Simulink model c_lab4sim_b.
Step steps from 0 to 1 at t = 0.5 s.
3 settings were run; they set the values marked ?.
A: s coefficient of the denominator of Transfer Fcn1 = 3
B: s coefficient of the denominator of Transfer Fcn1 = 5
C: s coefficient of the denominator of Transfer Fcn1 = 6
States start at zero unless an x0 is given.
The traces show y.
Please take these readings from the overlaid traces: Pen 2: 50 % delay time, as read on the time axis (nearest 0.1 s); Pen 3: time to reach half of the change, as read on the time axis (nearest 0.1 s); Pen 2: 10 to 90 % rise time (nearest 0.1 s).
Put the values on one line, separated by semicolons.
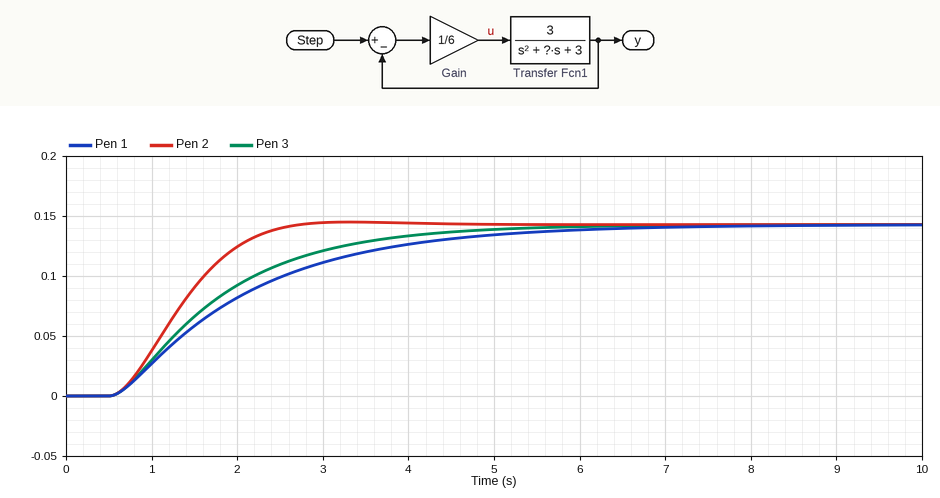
1.3 s; 1.6 s; 1.3 s
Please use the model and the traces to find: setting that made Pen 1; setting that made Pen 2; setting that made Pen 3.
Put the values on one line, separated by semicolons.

C; A; B
